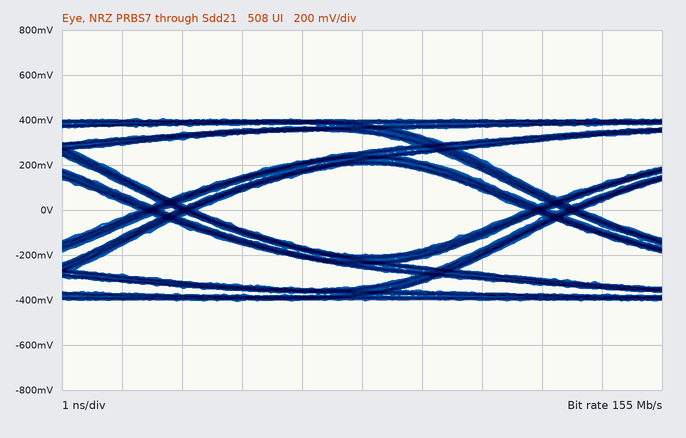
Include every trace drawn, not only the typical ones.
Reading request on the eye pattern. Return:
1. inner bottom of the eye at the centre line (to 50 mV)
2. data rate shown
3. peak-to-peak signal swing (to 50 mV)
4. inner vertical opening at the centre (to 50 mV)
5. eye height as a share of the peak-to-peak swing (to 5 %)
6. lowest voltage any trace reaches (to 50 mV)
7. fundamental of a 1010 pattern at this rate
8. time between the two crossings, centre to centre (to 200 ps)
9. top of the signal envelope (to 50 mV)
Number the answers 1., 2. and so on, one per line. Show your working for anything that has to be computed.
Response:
1. -200 mV
2. 155 Mb/s
3. 800 mV
4. 400 mV
5. 400 mV / 800 mV ≈ 50 %
6. -400 mV
7. 77.5 MHz
8. 6.4 ns
9. 400 mV
